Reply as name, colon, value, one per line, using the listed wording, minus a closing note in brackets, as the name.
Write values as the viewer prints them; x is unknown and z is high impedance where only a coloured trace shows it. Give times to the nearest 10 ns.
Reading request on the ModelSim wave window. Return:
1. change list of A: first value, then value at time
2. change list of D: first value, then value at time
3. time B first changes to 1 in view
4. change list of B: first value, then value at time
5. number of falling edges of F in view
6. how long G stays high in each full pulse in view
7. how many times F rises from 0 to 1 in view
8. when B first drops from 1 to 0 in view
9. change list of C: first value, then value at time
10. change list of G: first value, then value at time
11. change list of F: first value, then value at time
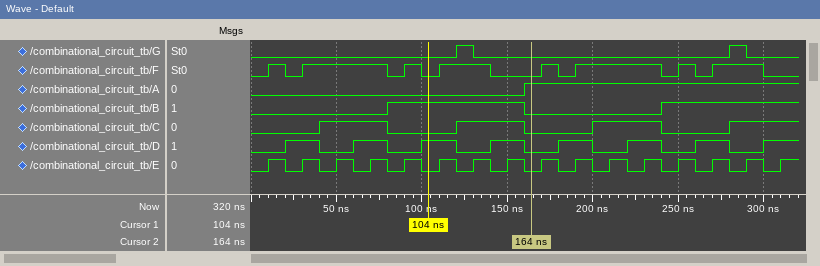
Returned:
change list of A: first value, then value at time: 0, 1 at 160 ns
change list of D: first value, then value at time: 0, 1 at 20 ns, 0 at 40 ns, 1 at 60 ns, 0 at 80 ns, 1 at 100 ns, 0 at 120 ns, 1 at 140 ns, 0 at 160 ns, 1 at 180 ns, 0 at 200 ns, 1 at 220 ns, 0 at 240 ns, 1 at 260 ns, 0 at 280 ns, 1 at 300 ns
time B first changes to 1 in view: 80 ns
change list of B: first value, then value at time: 0, 1 at 80 ns, 0 at 160 ns, 1 at 240 ns
number of falling edges of F in view: 8
how long G stays high in each full pulse in view: 10 ns, 10 ns
how many times F rises from 0 to 1 in view: 8
when B first drops from 1 to 0 in view: 160 ns
change list of C: first value, then value at time: 0, 1 at 40 ns, 0 at 80 ns, 1 at 120 ns, 0 at 160 ns, 1 at 200 ns, 0 at 240 ns, 1 at 280 ns
change list of G: first value, then value at time: 0, 1 at 120 ns, 0 at 130 ns, 1 at 280 ns, 0 at 290 ns
change list of F: first value, then value at time: 0, 1 at 10 ns, 0 at 20 ns, 1 at 30 ns, 0 at 80 ns, 1 at 90 ns, 0 at 100 ns, 1 at 110 ns, 0 at 140 ns, 1 at 170 ns, 0 at 180 ns, 1 at 190 ns, 0 at 240 ns, 1 at 250 ns, 0 at 260 ns, 1 at 270 ns, 0 at 300 ns
